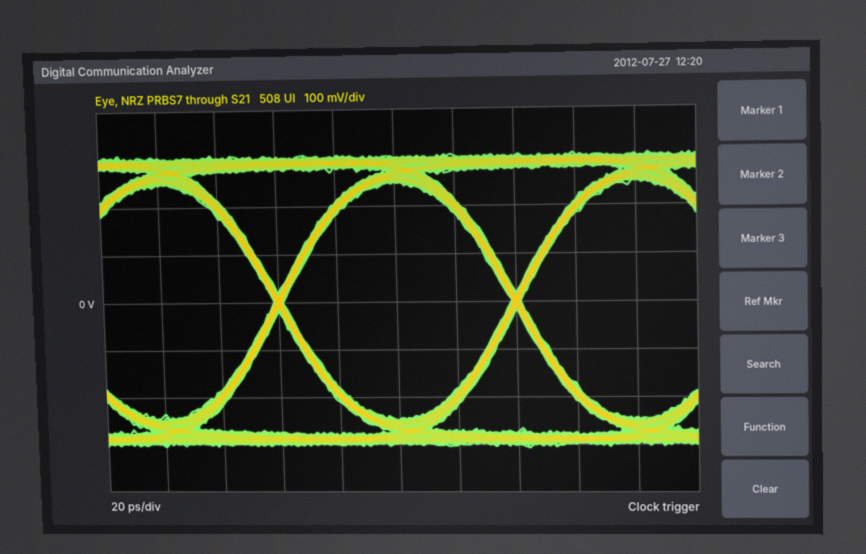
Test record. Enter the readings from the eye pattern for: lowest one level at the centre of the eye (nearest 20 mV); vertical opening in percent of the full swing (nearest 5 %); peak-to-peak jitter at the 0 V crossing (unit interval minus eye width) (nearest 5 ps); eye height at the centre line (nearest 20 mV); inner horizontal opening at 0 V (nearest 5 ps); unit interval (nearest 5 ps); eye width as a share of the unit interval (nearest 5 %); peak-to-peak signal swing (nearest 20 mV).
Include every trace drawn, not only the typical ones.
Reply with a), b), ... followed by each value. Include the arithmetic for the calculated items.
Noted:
a) 240 mV
b) 500 mV / 620 mV ≈ 80.6 %, so 80 % to the nearest 5 %
c) 5 ps
d) 500 mV
e) 75 ps
f) 80 ps
g) 75 ps / 80 ps ≈ 93.8 %, so 95 % to the nearest 5 %
h) 620 mV
